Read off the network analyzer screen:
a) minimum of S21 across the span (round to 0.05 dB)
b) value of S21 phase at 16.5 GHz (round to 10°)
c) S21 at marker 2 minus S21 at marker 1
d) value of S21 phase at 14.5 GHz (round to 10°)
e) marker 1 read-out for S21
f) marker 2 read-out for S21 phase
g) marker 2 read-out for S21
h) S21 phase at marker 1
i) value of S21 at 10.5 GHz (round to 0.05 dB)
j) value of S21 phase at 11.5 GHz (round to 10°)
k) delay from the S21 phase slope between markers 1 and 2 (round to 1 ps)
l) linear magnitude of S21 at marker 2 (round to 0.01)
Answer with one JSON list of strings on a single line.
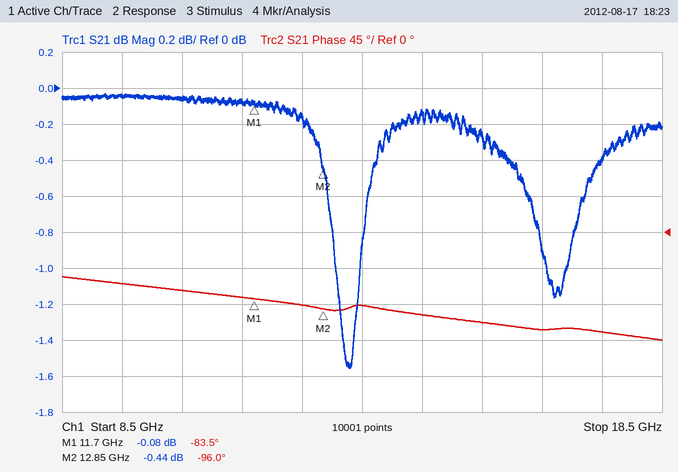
["-1.55 dB", "-120°", "-0.36 dB", "-100°", "-0.08 dB", "-96.0°", "-0.44 dB", "-83.5°", "-0.05 dB", "-80°", "30 ps", "0.95"]
